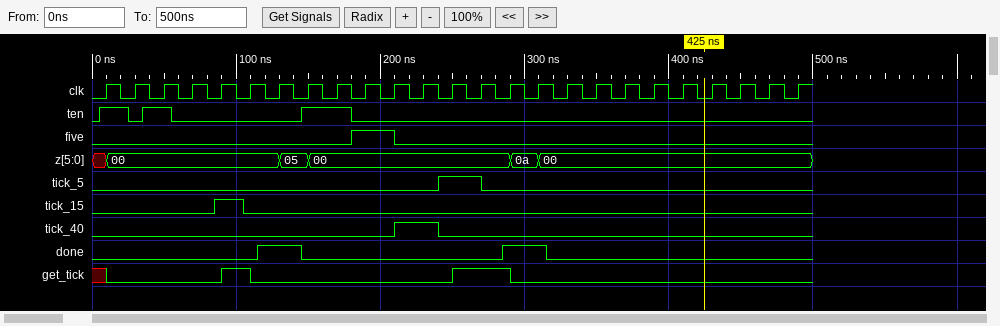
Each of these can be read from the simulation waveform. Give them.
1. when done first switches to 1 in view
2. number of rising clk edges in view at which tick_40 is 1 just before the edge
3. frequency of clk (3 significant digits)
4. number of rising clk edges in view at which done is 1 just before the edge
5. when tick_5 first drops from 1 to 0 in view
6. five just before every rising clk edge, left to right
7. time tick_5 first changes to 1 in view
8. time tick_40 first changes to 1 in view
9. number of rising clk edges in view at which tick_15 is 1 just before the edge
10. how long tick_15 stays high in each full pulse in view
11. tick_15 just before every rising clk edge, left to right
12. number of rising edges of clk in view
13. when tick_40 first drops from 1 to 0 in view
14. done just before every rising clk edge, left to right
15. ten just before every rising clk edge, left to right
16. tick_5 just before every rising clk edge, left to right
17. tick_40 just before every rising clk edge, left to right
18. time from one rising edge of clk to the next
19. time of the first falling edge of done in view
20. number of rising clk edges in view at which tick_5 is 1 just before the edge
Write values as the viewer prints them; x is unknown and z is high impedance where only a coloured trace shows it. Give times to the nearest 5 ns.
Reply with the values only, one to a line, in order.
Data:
115 ns
1
50.0 MHz
3
270 ns
0 0 0 0 0 0 0 0 0 1 1 0 0 0 0 0 0 0 0 0 0 0 0 0 0
240 ns
210 ns
1
20 ns
0 0 0 0 1 0 0 0 0 0 0 0 0 0 0 0 0 0 0 0 0 0 0 0 0
25
240 ns
0 0 0 0 0 0 1 0 0 0 0 0 0 0 1 1 0 0 0 0 0 0 0 0 0
1 0 1 0 0 0 0 1 1 0 0 0 0 0 0 0 0 0 0 0 0 0 0 0 0
0 0 0 0 0 0 0 0 0 0 0 0 1 1 0 0 0 0 0 0 0 0 0 0 0
0 0 0 0 0 0 0 0 0 0 0 1 0 0 0 0 0 0 0 0 0 0 0 0 0
20 ns
145 ns
2
